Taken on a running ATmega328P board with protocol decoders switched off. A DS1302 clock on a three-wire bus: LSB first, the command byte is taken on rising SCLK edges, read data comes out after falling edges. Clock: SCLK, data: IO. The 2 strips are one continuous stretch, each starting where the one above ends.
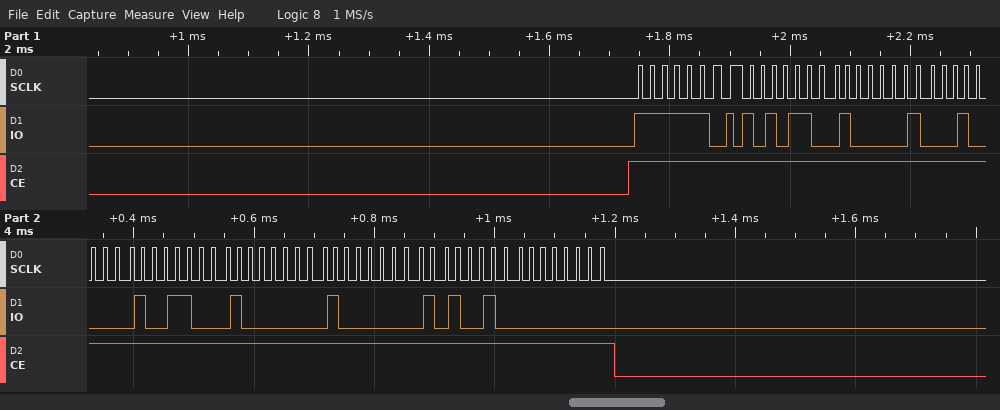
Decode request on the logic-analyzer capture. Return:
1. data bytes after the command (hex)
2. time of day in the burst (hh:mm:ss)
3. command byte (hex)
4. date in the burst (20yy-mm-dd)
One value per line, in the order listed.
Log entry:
35 41 04 19 01 01 25 00
04:41:35
0xBF
2025-01-19
